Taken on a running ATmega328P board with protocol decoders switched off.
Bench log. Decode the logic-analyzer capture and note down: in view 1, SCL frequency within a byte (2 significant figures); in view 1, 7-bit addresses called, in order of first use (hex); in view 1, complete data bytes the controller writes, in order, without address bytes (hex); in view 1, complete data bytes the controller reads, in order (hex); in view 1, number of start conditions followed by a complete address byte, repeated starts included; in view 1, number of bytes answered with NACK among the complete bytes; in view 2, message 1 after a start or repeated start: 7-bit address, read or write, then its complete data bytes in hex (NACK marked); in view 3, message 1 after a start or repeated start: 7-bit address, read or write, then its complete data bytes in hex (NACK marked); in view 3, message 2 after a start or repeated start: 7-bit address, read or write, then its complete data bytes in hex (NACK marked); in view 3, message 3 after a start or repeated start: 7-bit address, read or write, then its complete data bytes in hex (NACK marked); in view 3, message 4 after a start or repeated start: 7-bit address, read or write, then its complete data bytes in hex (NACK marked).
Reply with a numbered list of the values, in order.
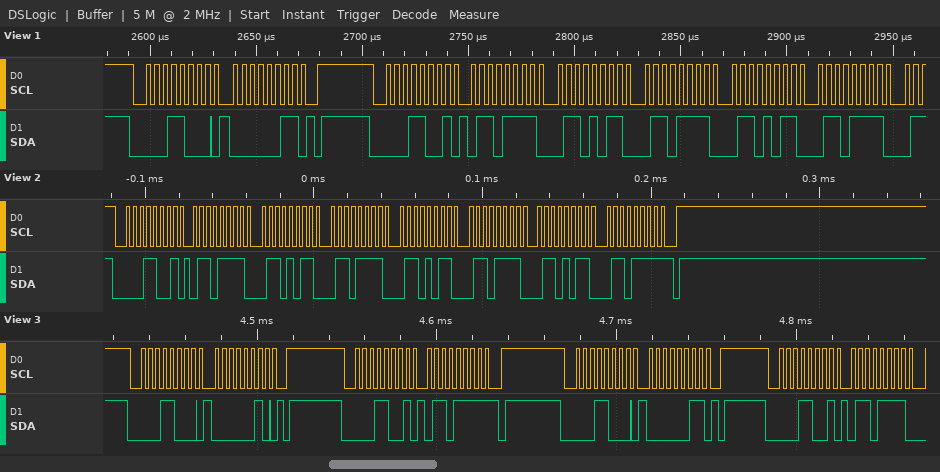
1. 250 kHz
2. 0x0C
3. 03
4. 6F 6B 6F 6B 6F
5. 2
6. 0
7. 0x0C read: 6F 6B 6F 6B 6F 6B 6F NACK
8. 0x0C write: 02
9. 0x0C read: 6F NACK
10. 0x0C write: 03
11. 0x0C read: 6F
